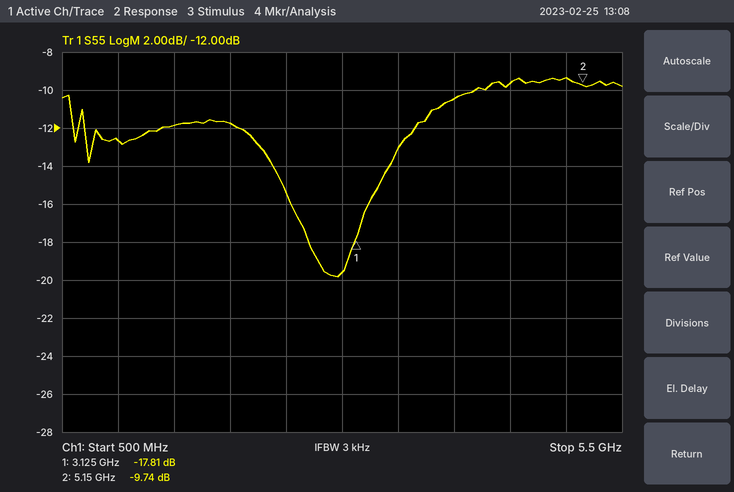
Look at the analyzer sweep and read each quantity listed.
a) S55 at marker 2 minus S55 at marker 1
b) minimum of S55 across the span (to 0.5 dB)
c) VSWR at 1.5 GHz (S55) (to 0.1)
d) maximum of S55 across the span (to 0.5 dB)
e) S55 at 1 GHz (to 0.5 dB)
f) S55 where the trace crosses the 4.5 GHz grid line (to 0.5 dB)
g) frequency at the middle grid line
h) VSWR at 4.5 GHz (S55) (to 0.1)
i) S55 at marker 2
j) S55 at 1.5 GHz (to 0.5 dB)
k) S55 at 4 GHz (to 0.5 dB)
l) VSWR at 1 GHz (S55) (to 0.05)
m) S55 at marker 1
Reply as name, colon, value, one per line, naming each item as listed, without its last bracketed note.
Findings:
S55 at marker 2 minus S55 at marker 1: 8.07 dB
minimum of S55 across the span: -20.0 dB
VSWR at 1.5 GHz (S55): 1.7
maximum of S55 across the span: -9.5 dB
S55 at 1 GHz: -12.5 dB
S55 where the trace crosses the 4.5 GHz grid line: -9.5 dB
frequency at the middle grid line: 3 GHz
VSWR at 4.5 GHz (S55): 2.0
S55 at marker 2: -9.74 dB
S55 at 1.5 GHz: -12.0 dB
S55 at 4 GHz: -10.5 dB
VSWR at 1 GHz (S55): 1.60
S55 at marker 1: -17.81 dB
